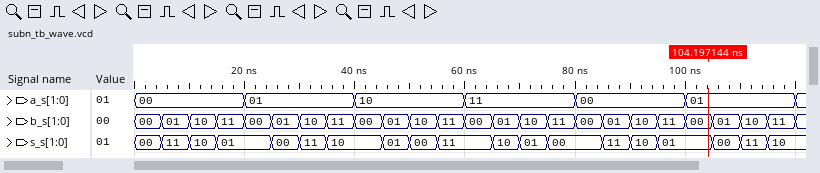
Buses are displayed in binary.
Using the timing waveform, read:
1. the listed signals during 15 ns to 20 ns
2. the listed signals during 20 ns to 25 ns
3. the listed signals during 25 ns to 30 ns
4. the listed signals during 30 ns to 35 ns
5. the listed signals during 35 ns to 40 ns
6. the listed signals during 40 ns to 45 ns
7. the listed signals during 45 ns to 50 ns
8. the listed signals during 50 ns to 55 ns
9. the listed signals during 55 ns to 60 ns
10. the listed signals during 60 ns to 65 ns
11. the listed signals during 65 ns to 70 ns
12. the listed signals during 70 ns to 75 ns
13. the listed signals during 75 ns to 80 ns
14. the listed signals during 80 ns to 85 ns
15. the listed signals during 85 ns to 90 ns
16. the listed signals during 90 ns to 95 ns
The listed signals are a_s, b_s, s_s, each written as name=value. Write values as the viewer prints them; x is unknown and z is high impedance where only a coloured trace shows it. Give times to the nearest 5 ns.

a_s=00, b_s=11, s_s=01
a_s=01, b_s=00, s_s=01
a_s=01, b_s=01, s_s=00
a_s=01, b_s=10, s_s=11
a_s=01, b_s=11, s_s=10
a_s=10, b_s=00, s_s=10
a_s=10, b_s=01, s_s=01
a_s=10, b_s=10, s_s=00
a_s=10, b_s=11, s_s=11
a_s=11, b_s=00, s_s=11
a_s=11, b_s=01, s_s=10
a_s=11, b_s=10, s_s=01
a_s=11, b_s=11, s_s=00
a_s=00, b_s=00, s_s=00
a_s=00, b_s=01, s_s=11
a_s=00, b_s=10, s_s=10
